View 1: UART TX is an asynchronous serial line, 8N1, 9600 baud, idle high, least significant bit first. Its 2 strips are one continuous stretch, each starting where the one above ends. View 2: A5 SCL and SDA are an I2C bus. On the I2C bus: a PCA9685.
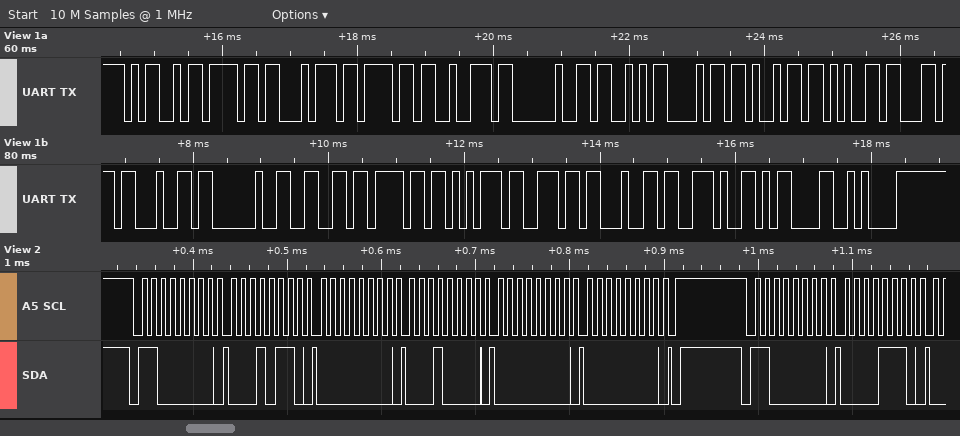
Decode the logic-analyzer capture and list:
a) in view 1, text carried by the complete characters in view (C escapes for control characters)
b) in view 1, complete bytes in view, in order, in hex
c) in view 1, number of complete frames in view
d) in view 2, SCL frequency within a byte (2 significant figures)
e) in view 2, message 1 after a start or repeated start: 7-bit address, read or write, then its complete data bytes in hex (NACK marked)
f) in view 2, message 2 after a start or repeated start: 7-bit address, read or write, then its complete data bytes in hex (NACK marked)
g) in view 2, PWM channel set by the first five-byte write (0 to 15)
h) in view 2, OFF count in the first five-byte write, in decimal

"Motor Shield found.\r\n"
4D 6F 74 6F 72 20 53 68 69 65 6C 64 20 66 6F 75 6E 64 2E 0D 0A
21
100 kHz
0x60 write: 16 00 10 00 00
0x60 write: 0E
4
0
